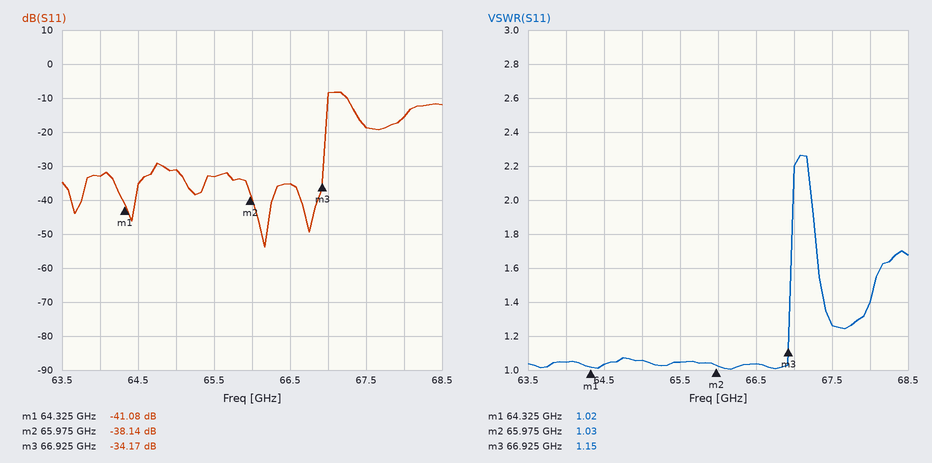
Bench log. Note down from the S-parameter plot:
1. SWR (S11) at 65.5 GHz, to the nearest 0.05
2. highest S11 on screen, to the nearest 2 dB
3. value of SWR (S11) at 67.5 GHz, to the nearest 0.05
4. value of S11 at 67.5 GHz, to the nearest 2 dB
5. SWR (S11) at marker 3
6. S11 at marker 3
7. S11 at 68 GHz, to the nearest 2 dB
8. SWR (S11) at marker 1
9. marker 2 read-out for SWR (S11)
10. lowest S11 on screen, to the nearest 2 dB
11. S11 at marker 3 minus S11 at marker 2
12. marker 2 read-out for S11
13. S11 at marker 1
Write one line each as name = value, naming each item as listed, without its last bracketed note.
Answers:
SWR (S11) at 65.5 GHz, to the nearest 0.05 = 1.05
highest S11 on screen, to the nearest 2 dB = -8 dB
value of SWR (S11) at 67.5 GHz, to the nearest 0.05 = 1.25
value of S11 at 67.5 GHz, to the nearest 2 dB = -18 dB
SWR (S11) at marker 3 = 1.15
S11 at marker 3 = -34.17 dB
S11 at 68 GHz, to the nearest 2 dB = -16 dB
SWR (S11) at marker 1 = 1.02
marker 2 read-out for SWR = 1.03
lowest S11 on screen, to the nearest 2 dB = -54 dB
S11 at marker 3 minus S11 at marker 2 = 3.97 dB
marker 2 read-out for S11 = -38.14 dB
S11 at marker 1 = -41.08 dB
